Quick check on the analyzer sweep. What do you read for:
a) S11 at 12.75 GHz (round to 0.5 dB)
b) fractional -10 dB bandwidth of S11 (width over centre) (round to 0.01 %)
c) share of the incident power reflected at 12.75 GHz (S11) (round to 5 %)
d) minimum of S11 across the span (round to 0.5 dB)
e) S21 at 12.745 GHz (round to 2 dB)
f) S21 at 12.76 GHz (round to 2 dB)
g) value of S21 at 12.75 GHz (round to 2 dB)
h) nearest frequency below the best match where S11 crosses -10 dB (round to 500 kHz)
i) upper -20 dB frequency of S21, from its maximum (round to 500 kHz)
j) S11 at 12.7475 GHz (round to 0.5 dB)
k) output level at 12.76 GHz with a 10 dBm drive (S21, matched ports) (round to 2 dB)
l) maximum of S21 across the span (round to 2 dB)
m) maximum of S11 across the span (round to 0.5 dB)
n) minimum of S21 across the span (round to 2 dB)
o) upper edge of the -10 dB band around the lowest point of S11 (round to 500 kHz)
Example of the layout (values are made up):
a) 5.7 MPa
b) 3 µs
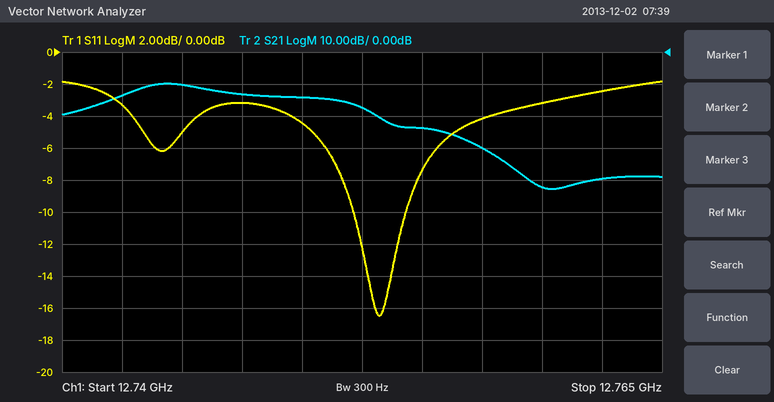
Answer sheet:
a) -4.5 dB
b) 0.02 %
c) 35 %
d) -16.5 dB
e) -10 dB
f) -42 dB
g) -14 dB
h) 12.7520 GHz
i) 12.7575 GHz
j) -3.0 dB
k) -32 dBm
l) -10 dB
m) -2.0 dB
n) -42 dB
o) 12.7545 GHz
